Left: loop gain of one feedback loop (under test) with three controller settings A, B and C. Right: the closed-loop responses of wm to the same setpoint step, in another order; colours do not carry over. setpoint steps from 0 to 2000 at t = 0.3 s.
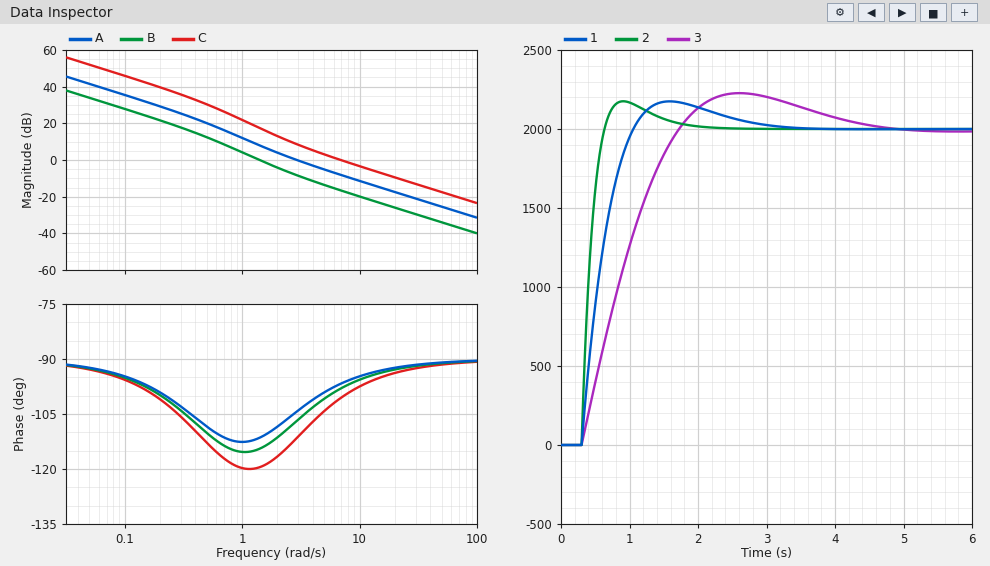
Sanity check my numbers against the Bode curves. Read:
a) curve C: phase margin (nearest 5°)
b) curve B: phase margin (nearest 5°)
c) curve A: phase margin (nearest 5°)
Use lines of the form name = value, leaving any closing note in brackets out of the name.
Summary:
curve C: phase margin = 80°
curve B: phase margin = 65°
curve A: phase margin = 75°
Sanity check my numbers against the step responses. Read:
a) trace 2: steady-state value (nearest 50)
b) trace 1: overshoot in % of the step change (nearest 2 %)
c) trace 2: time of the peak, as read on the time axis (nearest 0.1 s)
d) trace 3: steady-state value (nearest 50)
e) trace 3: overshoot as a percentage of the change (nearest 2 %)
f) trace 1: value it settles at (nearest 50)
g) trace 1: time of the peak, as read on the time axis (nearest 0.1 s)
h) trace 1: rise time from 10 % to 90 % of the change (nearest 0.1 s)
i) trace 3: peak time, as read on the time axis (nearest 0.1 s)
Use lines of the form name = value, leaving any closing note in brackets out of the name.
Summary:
trace 2: steady-state value = 2000
trace 1: overshoot in % of the step change = 8 %
trace 2: time of the peak, as read on the time axis = 0.9 s
trace 3: steady-state value = 2000
trace 3: overshoot as a percentage of the change = 12 %
trace 1: value it settles at = 2000
trace 1: time of the peak, as read on the time axis = 1.6 s
trace 1: rise time from 10 % to 90 % of the change = 0.5 s
trace 3: peak time, as read on the time axis = 2.6 s
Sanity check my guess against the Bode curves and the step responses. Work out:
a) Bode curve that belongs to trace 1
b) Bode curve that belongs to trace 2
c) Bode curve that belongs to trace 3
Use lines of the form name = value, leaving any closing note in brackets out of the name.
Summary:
Bode curve that belongs to trace 1 = A
Bode curve that belongs to trace 2 = C
Bode curve that belongs to trace 3 = B
